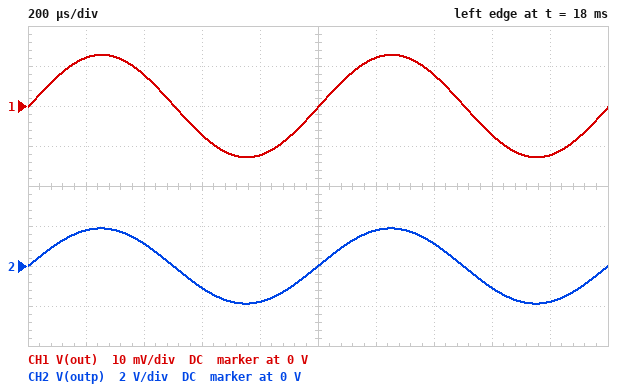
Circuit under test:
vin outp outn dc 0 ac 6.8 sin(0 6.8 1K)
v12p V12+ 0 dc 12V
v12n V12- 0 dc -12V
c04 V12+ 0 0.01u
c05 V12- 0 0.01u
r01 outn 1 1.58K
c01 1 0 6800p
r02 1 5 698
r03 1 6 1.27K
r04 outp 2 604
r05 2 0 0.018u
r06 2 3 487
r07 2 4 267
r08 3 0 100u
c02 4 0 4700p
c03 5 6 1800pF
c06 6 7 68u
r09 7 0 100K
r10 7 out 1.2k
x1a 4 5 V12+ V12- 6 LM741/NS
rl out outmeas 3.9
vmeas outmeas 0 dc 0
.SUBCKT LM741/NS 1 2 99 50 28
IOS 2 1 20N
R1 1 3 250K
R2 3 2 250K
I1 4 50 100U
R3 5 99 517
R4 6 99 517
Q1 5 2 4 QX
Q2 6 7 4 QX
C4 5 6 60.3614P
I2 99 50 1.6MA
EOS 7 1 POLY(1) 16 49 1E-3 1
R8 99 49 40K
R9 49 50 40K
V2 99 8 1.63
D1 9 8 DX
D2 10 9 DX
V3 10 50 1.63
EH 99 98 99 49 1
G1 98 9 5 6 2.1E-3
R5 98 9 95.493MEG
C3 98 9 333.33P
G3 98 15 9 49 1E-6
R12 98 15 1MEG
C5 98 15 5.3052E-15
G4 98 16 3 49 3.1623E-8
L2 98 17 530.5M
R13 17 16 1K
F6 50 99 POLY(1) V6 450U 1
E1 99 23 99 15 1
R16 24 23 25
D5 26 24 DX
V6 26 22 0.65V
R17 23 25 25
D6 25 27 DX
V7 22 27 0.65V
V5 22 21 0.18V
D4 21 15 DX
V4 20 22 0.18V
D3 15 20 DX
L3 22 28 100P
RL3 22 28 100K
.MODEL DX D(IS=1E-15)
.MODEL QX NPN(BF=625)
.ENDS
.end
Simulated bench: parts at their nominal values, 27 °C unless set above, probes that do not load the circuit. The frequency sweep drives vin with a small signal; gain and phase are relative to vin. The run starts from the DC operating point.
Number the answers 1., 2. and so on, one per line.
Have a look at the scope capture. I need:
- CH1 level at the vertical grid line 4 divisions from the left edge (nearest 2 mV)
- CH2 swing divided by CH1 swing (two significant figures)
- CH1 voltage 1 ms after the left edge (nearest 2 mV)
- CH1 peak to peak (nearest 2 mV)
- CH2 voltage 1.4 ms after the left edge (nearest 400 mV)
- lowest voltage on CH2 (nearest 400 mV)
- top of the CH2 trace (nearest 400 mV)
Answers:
1. -12 mV
2. 150
3. 0 V
4. 26 mV
5. 1.2 V
6. -2.0 V
7. 2.0 V
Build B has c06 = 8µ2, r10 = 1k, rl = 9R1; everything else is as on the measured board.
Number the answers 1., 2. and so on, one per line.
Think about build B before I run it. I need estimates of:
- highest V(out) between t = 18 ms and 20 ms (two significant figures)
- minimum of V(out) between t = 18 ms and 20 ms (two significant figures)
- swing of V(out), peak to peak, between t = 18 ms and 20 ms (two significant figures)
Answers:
1. 36 mV
2. -36 mV
3. 71 mV
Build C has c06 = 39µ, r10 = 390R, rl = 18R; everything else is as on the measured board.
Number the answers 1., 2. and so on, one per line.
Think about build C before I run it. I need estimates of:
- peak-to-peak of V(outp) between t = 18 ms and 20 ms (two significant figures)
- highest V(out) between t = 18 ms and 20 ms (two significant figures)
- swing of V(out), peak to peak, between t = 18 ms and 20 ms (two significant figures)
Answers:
1. 3.8 V
2. 170 mV
3. 350 mV
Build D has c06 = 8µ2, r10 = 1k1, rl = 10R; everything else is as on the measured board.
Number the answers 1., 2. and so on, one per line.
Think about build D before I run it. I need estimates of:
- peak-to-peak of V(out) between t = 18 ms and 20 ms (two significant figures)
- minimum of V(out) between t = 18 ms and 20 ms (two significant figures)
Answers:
1. 71 mV
2. -36 mV
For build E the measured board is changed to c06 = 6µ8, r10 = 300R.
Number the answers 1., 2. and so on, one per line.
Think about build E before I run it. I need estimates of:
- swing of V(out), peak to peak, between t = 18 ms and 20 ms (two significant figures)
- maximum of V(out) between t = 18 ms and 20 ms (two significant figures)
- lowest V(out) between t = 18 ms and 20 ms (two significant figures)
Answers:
1. 100 mV
2. 51 mV
3. -51 mV
